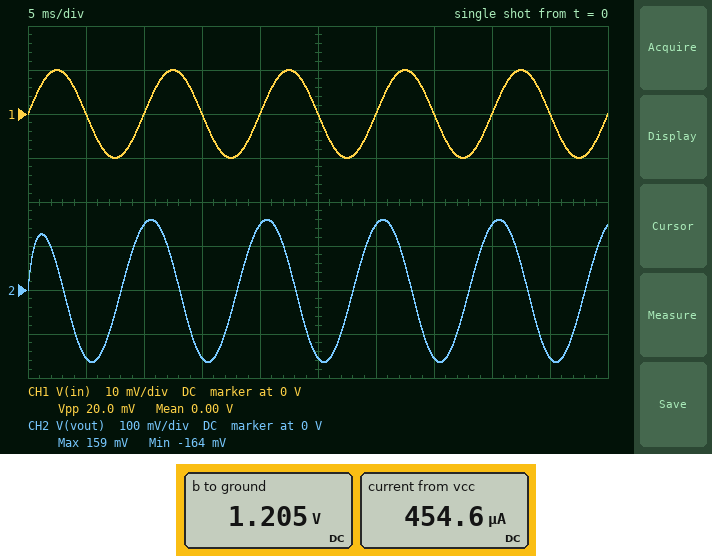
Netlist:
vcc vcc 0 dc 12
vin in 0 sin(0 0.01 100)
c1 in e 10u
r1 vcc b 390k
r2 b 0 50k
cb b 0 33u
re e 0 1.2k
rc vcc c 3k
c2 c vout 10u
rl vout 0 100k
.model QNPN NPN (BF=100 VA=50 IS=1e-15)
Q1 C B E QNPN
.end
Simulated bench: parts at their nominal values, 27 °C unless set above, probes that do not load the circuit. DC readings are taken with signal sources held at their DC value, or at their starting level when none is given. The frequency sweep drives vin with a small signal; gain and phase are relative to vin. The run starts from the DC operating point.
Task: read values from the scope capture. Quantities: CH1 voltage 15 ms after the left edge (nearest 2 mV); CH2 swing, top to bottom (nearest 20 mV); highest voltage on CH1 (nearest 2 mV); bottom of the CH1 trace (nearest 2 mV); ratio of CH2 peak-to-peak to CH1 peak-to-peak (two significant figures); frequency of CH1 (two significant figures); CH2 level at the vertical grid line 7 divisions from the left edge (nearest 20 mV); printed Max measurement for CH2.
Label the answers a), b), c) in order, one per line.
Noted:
a) 0 V
b) 320 mV
c) 10 mV
d) -10 mV
e) 16
f) 100 Hz
g) -160 mV
h) 159 mV
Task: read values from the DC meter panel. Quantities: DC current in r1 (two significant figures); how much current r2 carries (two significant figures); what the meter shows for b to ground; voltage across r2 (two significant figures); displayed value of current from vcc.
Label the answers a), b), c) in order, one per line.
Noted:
a) 28 µA
b) 24 µA
c) 1.205 V
d) 1.2 V
e) 454.6 µA
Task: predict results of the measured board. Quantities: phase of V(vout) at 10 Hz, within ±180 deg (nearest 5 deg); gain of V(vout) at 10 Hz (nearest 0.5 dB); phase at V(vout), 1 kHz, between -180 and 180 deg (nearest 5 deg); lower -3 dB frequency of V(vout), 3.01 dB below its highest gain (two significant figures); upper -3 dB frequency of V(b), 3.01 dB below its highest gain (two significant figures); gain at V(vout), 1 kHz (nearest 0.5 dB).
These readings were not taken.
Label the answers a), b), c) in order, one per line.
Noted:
a) 90 deg
b) 4.5 dB
c) 15 deg
d) 270 Hz
e) 270 Hz
f) 33.0 dB
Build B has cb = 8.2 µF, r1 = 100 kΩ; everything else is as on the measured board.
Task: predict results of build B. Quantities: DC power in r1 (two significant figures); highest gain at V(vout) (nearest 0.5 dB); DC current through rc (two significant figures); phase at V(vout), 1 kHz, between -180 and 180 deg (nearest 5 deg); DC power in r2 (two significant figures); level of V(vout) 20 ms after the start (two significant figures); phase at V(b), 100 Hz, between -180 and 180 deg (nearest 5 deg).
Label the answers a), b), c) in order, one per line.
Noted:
a) 750 µW
b) 46.5 dB
c) 2.1 mA
d) 50 deg
e) 220 µW
f) 180 mV
g) -5 deg
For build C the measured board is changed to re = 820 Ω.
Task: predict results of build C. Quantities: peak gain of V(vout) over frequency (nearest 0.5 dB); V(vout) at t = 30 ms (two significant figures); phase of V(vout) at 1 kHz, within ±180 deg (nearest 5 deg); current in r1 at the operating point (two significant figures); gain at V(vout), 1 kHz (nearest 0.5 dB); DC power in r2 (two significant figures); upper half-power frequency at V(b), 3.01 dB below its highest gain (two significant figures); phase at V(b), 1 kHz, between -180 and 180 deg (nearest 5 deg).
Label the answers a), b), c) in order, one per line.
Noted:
a) 35.5 dB
b) 160 mV
c) 20 deg
d) 28 µA
e) 35.0 dB
f) 27 µW
g) 360 Hz
h) -70 deg
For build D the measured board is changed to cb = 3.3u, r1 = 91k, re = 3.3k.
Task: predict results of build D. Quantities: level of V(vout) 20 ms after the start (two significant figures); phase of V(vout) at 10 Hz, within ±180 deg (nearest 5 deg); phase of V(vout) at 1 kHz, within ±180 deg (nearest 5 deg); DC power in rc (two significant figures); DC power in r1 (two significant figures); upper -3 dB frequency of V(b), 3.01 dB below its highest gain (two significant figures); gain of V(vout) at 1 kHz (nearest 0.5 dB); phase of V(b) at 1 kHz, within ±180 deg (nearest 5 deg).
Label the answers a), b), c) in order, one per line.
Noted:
a) 170 mV
b) 90 deg
c) 30 deg
d) 2.9 mW
e) 710 µW
f) 600 Hz
g) 39.0 dB
h) -60 deg
